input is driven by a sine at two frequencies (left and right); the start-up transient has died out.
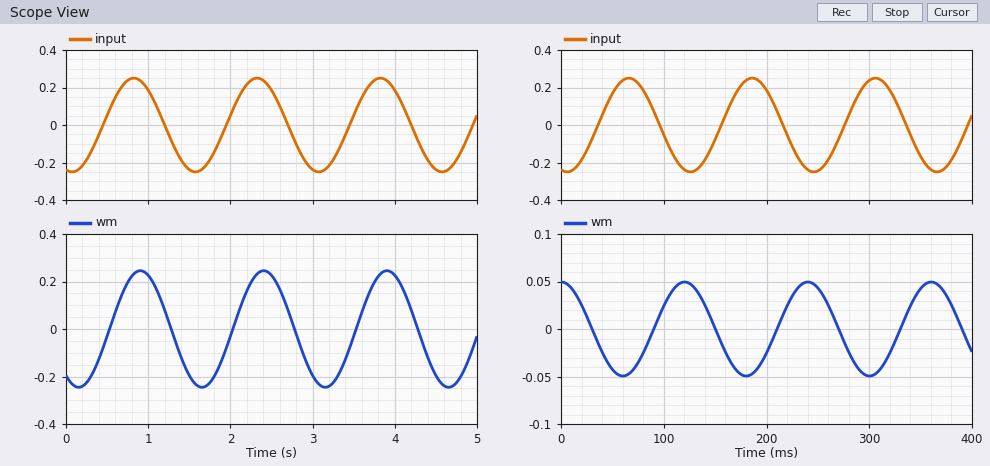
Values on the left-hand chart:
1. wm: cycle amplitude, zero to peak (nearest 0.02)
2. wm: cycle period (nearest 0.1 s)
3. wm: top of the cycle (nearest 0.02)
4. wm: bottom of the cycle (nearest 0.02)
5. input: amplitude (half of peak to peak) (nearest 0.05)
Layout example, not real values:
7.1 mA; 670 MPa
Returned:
0.24; 1.5 s; 0.24; -0.24; 0.25
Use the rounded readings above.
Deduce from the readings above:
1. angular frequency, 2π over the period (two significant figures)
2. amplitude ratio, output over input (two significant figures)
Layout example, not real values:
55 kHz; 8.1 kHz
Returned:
4.2 rad/s; 0.96
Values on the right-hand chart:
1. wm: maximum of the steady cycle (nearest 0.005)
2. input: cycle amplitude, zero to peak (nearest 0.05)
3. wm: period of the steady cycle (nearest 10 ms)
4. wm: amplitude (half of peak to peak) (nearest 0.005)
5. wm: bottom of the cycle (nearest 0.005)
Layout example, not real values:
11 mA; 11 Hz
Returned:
0.050; 0.25; 120 ms; 0.050; -0.050
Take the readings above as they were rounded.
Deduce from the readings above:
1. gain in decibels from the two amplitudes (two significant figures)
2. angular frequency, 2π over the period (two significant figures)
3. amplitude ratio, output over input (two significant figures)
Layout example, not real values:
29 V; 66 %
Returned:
-14 dB; 0.052 rad/ms; 0.20
